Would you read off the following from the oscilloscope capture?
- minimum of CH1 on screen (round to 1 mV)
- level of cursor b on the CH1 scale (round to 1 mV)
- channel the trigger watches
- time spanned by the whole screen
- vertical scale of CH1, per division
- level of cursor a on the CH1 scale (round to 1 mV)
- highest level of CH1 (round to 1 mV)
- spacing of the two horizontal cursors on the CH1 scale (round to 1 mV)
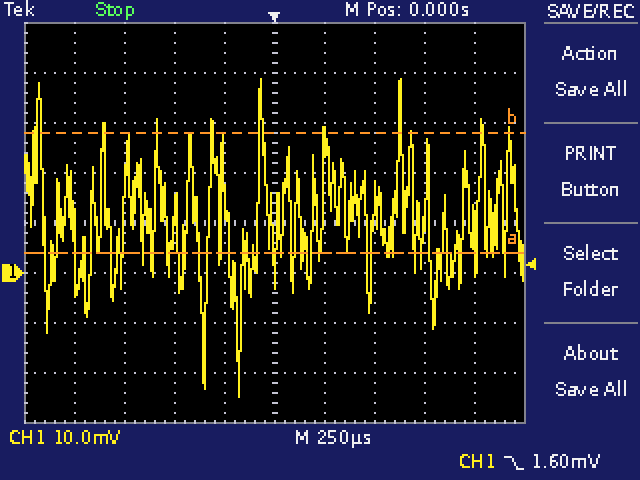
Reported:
-25 mV
28 mV
CH1
2.5 ms
10 mV
4 mV
39 mV
24 mV
